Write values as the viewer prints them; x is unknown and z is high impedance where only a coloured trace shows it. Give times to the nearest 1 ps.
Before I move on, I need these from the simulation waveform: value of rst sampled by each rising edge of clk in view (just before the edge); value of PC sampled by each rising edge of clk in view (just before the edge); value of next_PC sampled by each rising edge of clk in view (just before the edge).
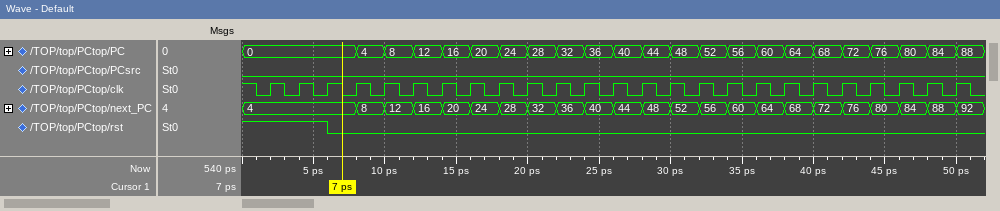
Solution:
1 1 1 0 0 0 0 0 0 0 0 0 0 0 0 0 0 0 0 0 0 0 0 0 0
0, 0, 0, 0, 4, 8, 12, 16, 20, 24, 28, 32, 36, 40, 44, 48, 52, 56, 60, 64, 68, 72, 76, 80, 84
4, 4, 4, 4, 8, 12, 16, 20, 24, 28, 32, 36, 40, 44, 48, 52, 56, 60, 64, 68, 72, 76, 80, 84, 88
